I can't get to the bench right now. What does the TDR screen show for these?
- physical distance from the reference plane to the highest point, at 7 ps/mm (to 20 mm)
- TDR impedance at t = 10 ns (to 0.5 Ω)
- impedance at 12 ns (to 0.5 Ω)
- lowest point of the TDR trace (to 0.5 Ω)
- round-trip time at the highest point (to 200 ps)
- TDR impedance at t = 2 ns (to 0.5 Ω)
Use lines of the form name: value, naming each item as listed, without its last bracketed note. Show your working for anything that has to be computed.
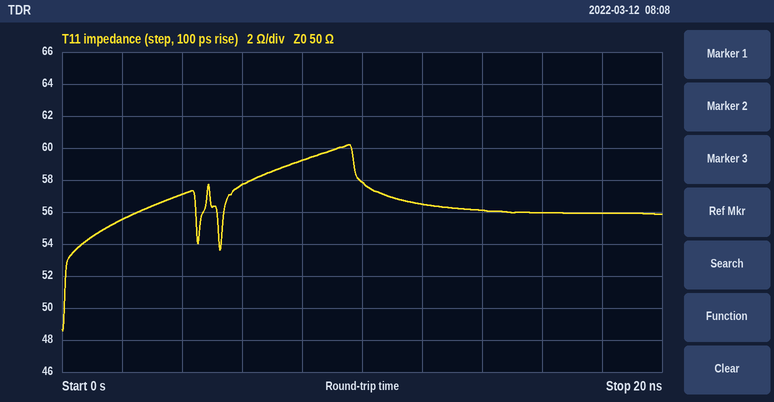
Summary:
physical distance from the reference plane to the highest point, at 7 ps/mm: 9.6 ns / 2 / 7 ps/mm ≈ 686 mm, so 680 mm to the nearest 20 mm
TDR impedance at t = 10 ns: 58.0 Ω
impedance at 12 ns: 56.5 Ω
lowest point of the TDR trace: 48.5 Ω
round-trip time at the highest point: 9.6 ns
TDR impedance at t = 2 ns: 55.5 Ω
